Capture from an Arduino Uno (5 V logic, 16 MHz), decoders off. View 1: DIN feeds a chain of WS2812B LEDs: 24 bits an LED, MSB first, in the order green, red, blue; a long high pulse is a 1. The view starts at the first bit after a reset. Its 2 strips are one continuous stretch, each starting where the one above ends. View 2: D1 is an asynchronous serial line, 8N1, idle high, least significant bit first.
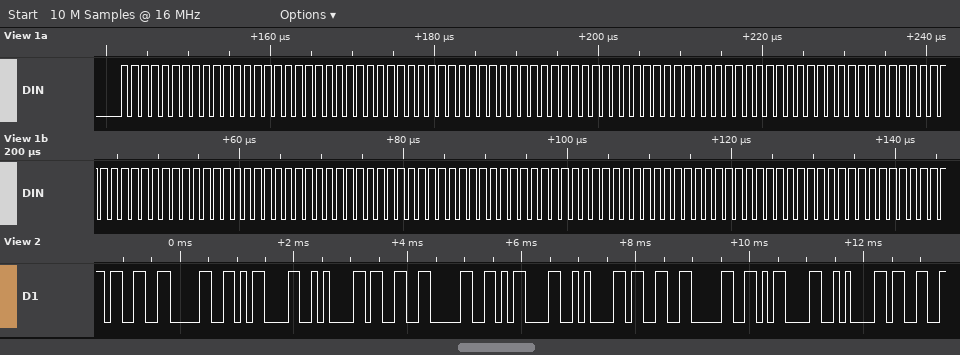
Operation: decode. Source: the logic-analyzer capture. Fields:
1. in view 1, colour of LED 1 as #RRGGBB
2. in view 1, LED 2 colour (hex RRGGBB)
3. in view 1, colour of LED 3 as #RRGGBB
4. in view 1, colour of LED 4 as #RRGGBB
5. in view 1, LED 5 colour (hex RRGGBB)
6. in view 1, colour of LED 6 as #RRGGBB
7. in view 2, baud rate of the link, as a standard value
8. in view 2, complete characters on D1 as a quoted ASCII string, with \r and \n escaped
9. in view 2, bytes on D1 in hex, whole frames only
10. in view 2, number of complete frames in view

#FFFFFF
#FFFFFF
#FFFFFF
#FFFFFF
#FFFFFF
#FFFFFF
9600 baud
"30\r\n30\r\n30\r\n3"
33 30 0D 0A 33 30 0D 0A 33 30 0D 0A 33
13
